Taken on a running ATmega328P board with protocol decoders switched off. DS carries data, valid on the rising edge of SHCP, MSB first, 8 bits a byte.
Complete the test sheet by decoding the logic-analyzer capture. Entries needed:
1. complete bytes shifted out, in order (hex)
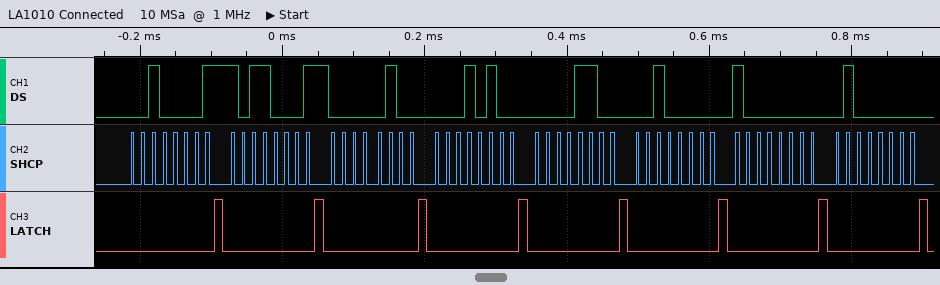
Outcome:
21 B1 04 14 0C 20 80 40
